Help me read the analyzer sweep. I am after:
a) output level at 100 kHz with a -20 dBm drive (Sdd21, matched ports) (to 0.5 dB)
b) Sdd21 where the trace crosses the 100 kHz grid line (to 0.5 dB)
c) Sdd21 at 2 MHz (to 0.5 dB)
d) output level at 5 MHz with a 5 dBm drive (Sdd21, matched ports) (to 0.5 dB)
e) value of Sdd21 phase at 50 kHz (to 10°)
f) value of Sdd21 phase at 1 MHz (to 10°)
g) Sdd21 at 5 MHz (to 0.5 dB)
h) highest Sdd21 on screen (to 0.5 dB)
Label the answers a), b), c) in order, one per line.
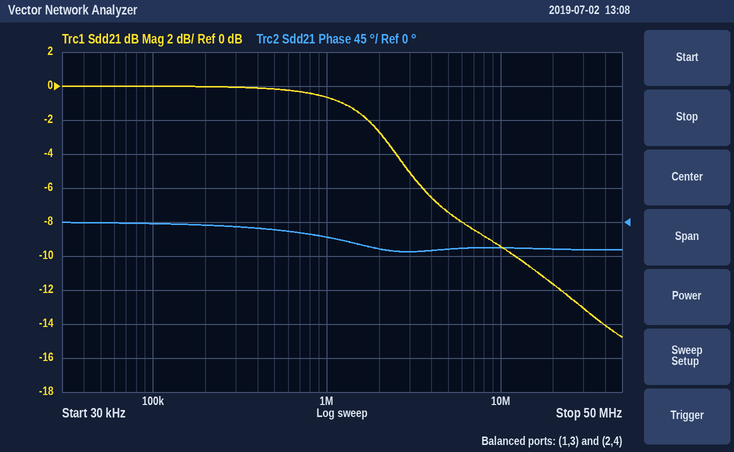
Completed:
a) -20.0 dBm
b) 0.0 dB
c) -2.5 dB
d) -2.5 dBm
e) 0°
f) -20°
g) -7.5 dB
h) 0.0 dB
